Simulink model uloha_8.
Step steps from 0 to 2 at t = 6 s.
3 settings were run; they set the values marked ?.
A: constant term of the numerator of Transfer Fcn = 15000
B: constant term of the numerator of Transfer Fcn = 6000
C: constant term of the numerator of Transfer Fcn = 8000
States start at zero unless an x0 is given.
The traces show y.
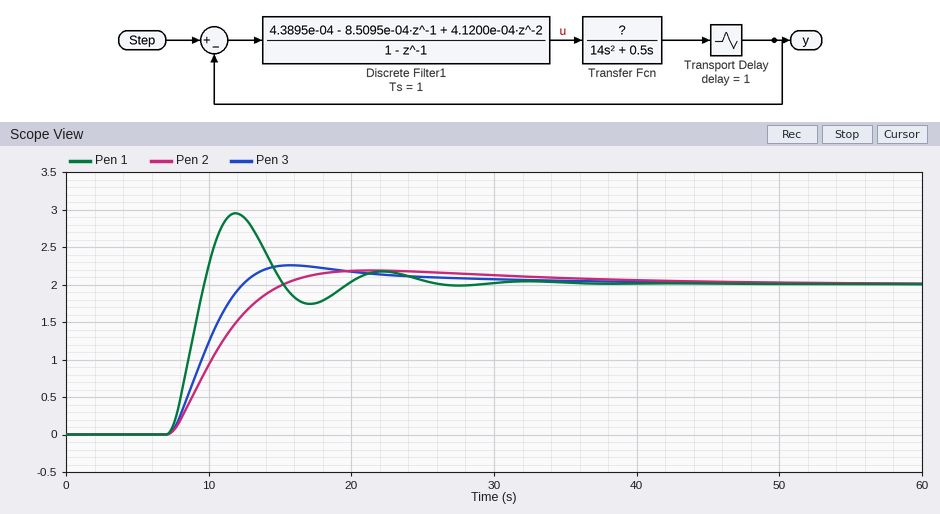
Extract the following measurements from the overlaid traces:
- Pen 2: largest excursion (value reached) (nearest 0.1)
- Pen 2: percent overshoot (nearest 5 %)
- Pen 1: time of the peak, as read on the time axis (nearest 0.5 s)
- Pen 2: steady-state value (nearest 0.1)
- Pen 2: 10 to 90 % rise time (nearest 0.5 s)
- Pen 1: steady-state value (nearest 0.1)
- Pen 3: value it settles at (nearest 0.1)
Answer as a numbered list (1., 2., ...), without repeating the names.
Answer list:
1. 2.2
2. 10 %
3. 12.0 s
4. 2.0
5. 5.5 s
6. 2.0
7. 2.0
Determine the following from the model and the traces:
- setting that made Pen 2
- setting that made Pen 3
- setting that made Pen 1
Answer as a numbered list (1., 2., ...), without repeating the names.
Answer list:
1. B
2. C
3. A
